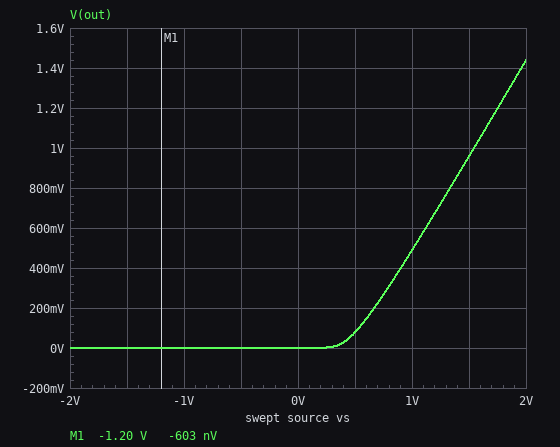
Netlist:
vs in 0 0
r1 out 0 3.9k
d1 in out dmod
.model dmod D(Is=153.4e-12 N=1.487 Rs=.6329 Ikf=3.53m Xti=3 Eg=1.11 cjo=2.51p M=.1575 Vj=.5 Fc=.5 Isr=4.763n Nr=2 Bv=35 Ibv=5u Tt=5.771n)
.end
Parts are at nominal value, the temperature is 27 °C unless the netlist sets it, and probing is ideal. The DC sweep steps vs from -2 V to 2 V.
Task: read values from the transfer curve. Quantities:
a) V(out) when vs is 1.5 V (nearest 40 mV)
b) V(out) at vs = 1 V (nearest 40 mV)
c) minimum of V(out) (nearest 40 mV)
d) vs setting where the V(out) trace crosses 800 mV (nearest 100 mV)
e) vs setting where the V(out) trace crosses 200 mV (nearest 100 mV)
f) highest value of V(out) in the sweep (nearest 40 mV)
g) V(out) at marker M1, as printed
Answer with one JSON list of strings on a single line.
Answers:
["960 mV", "480 mV", "0 V", "1.3 V", "700 mV", "1.44 V", "-603 nV"]
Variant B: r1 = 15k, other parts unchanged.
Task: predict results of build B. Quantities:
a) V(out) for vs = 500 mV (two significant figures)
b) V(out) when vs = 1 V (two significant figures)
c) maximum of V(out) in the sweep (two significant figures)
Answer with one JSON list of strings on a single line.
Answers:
["120 mV", "550 mV", "1.5 V"]
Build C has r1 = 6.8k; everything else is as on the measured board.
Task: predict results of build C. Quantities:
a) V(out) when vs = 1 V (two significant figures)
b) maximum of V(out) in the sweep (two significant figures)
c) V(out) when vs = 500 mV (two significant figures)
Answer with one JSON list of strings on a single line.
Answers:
["510 mV", "1.5 V", "95 mV"]
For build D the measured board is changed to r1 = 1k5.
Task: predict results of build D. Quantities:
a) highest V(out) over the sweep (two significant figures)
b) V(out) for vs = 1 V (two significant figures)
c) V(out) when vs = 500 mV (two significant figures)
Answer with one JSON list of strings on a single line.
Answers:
["1.4 V", "450 mV", "51 mV"]
